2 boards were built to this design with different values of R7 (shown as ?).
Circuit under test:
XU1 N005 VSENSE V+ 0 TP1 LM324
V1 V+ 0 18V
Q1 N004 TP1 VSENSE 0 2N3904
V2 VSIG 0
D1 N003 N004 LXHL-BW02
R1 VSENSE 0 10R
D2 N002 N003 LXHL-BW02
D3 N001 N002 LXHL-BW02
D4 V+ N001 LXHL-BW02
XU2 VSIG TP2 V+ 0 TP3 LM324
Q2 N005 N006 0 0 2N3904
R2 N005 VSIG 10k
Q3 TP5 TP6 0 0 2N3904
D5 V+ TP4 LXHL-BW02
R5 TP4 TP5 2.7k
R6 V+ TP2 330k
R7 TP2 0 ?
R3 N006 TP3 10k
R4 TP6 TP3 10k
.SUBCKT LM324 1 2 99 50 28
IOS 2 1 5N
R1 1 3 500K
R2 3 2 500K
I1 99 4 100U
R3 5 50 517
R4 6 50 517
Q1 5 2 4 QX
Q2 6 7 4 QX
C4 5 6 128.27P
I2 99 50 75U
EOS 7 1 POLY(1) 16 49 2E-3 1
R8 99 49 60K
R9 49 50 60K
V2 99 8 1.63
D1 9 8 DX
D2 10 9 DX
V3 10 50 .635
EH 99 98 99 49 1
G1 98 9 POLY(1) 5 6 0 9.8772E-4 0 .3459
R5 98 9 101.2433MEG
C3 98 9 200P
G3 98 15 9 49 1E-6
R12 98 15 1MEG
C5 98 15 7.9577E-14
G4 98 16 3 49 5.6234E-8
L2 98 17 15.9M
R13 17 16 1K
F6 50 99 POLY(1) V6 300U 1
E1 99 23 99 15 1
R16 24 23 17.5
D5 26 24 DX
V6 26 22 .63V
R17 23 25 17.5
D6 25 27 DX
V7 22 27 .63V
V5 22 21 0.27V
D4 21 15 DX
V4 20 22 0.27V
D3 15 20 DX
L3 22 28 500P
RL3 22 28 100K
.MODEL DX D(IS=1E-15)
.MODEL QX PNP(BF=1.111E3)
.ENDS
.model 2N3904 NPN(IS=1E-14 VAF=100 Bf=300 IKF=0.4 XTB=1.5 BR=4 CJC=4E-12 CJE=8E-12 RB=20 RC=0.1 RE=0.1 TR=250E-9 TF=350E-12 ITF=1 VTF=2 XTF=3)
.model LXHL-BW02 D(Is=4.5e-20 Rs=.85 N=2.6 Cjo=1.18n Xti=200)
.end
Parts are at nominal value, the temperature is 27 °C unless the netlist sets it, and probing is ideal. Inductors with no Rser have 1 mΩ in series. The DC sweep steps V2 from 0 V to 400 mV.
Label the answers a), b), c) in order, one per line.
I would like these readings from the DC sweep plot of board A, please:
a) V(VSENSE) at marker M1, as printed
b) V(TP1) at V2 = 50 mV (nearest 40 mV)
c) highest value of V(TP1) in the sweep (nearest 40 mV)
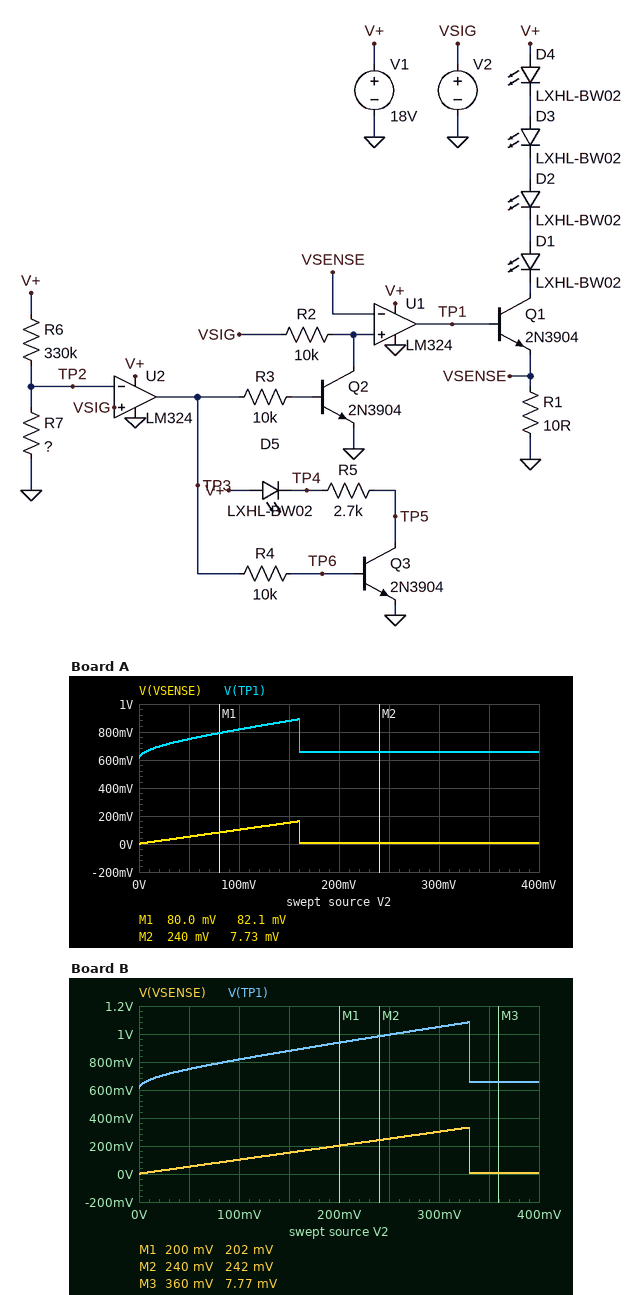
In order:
a) 82.1 mV
b) 760 mV
c) 880 mV
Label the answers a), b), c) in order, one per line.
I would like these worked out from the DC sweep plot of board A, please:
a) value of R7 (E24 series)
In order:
a) 3 kΩ
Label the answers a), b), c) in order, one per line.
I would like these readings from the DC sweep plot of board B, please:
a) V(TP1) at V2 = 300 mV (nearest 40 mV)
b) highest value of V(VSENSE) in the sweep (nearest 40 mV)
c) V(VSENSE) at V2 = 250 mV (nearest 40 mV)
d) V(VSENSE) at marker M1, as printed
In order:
a) 1.04 V
b) 320 mV
c) 240 mV
d) 202 mV
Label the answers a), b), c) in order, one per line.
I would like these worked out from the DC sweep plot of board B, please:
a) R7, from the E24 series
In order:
a) 6.2 kΩ
